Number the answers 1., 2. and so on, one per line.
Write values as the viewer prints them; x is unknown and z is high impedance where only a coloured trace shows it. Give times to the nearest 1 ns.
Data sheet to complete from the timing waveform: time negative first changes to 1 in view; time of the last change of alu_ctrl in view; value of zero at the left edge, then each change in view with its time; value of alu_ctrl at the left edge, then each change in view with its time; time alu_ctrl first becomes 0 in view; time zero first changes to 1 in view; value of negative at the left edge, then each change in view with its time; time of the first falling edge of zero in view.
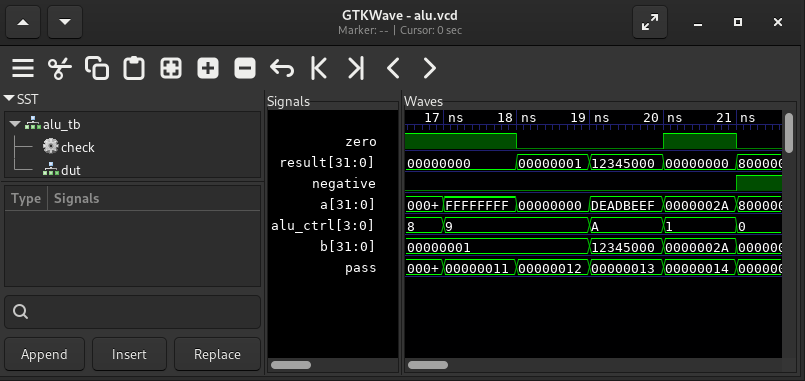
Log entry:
1. 21 ns
2. 21 ns
3. 1, 0 at 18 ns, 1 at 20 ns, 0 at 21 ns
4. 8, 9 at 17 ns, A at 19 ns, 1 at 20 ns, 0 at 21 ns
5. 21 ns
6. 20 ns
7. 0, 1 at 21 ns
8. 18 ns
